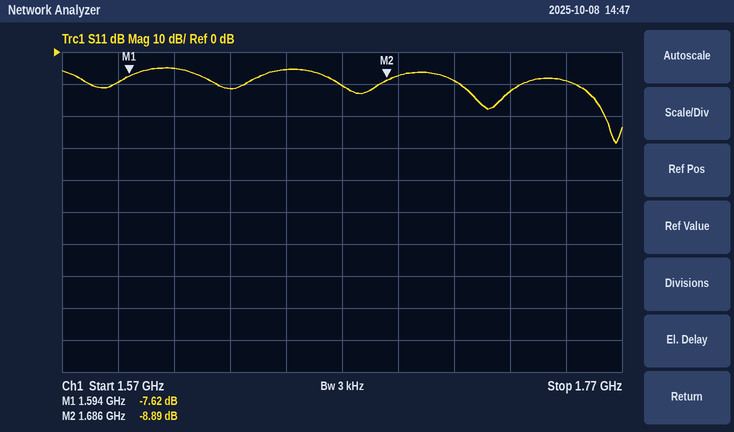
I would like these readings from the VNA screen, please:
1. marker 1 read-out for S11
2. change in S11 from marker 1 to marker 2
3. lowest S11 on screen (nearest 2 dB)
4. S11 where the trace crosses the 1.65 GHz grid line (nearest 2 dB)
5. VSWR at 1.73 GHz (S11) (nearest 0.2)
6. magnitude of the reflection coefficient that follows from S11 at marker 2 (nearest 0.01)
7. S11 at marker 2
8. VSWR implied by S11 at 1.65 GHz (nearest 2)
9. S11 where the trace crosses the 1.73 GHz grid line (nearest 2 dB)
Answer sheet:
-7.62 dB
-1.27 dB
-28 dB
-6 dB
1.6
0.36
-8.89 dB
4
-12 dB
